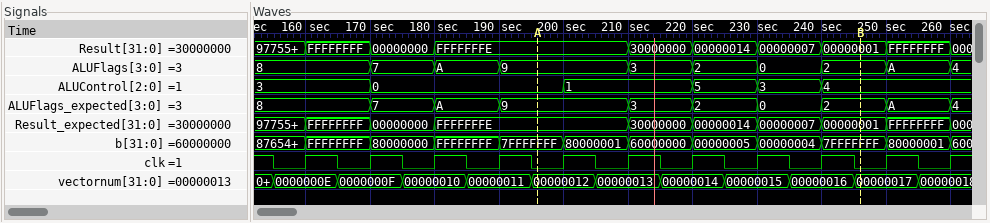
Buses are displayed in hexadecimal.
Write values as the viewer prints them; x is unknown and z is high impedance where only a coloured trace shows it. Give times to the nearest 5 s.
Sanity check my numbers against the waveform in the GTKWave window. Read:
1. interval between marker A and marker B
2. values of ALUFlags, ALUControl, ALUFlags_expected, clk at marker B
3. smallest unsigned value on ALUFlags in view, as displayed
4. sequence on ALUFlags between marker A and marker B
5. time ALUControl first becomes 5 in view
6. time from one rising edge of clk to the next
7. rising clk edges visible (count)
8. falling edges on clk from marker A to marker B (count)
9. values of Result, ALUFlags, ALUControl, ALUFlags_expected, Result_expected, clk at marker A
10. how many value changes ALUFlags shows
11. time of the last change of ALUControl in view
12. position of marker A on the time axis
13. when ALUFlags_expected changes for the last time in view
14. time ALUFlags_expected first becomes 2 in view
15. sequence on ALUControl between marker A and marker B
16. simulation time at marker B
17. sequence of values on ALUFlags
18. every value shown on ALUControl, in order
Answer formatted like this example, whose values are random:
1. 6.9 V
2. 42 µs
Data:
1. 50 s
2. ALUFlags=2, ALUControl=4, ALUFlags_expected=2, clk=0
3. 0
4. 9, 3, 2, 0, 2
5. 220 s
6. 10 s
7. 11
8. 5
9. Result=FFFFFFFE, ALUFlags=9, ALUControl=0, ALUFlags_expected=9, Result_expected=FFFFFFFE, clk=0
10. 9
11. 240 s
12. 195 s
13. 260 s
14. 220 s
15. 0, 1, 5, 3, 4
16. 245 s
17. 8, 7, A, 9, 3, 2, 0, 2, A, 4
18. 3, 0, 1, 5, 3, 4
